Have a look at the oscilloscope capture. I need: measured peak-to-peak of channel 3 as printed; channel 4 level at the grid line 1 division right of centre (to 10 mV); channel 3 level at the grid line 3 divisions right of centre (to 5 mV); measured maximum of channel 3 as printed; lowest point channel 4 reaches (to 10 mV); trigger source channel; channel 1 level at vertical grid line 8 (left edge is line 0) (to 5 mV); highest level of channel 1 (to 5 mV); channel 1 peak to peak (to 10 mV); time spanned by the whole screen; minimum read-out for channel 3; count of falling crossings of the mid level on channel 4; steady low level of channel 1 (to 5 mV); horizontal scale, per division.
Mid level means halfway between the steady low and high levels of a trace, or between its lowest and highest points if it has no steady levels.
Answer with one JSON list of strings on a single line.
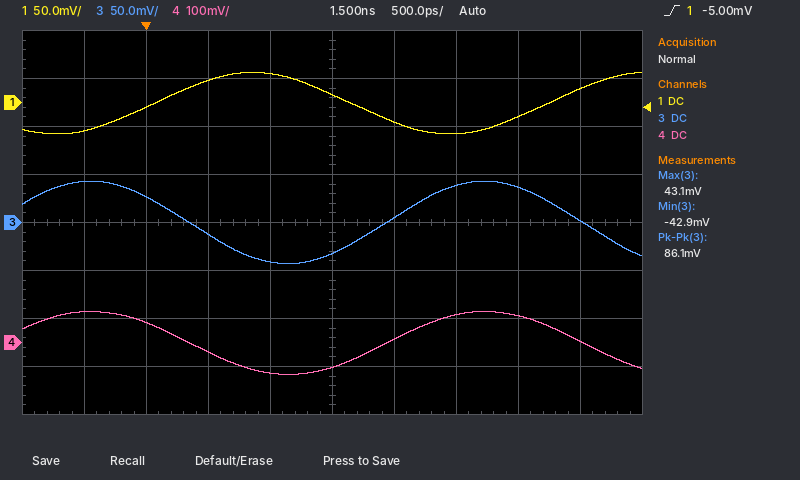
["86.1 mV", "10 mV", "35 mV", "43.1 mV", "-70 mV", "channel 1", "-15 mV", "30 mV", "60 mV", "5 ns", "-42.9 mV", "2", "-30 mV", "500 ps"]
